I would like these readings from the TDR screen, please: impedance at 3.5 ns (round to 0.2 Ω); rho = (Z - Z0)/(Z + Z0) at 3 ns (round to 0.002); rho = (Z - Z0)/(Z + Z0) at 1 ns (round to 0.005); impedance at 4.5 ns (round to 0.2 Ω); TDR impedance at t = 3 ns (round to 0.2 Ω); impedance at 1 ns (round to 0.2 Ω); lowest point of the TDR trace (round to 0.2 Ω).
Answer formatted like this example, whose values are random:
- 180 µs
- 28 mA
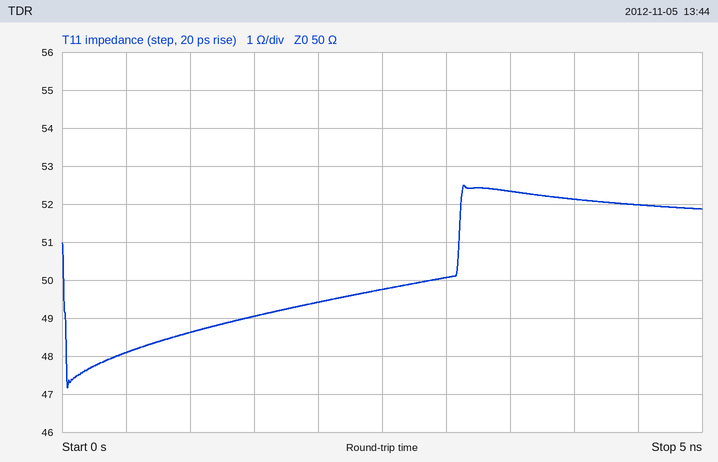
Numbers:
- 52.4 Ω
- 0.000
- -0.015
- 52.0 Ω
- 50.0 Ω
- 48.6 Ω
- 47.2 Ω
